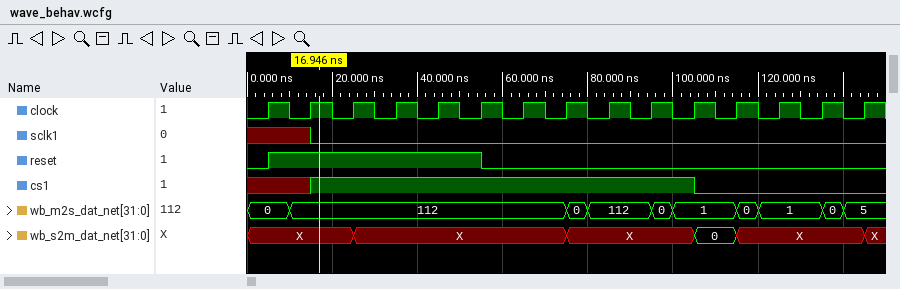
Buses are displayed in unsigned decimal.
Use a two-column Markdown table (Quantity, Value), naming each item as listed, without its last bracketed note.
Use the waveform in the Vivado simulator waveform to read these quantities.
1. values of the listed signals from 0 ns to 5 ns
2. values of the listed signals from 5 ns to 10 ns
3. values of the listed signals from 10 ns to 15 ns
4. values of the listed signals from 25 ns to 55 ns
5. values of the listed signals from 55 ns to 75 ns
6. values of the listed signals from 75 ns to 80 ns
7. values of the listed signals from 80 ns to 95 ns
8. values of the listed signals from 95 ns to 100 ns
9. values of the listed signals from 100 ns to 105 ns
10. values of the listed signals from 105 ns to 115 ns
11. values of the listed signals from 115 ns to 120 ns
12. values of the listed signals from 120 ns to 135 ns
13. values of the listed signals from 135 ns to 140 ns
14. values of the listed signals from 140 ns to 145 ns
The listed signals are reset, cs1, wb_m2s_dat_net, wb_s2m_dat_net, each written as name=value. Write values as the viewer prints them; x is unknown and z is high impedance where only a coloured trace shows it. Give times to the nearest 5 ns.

| Quantity | Value |
|---|---|
| values of the listed signals from 0 ns to 5 ns | reset=0, cs1=x, wb_m2s_dat_net=0, wb_s2m_dat_net=X |
| values of the listed signals from 5 ns to 10 ns | reset=1, cs1=x, wb_m2s_dat_net=0, wb_s2m_dat_net=X |
| values of the listed signals from 10 ns to 15 ns | reset=1, cs1=x, wb_m2s_dat_net=112, wb_s2m_dat_net=X |
| values of the listed signals from 25 ns to 55 ns | reset=1, cs1=1, wb_m2s_dat_net=112, wb_s2m_dat_net=X |
| values of the listed signals from 55 ns to 75 ns | reset=0, cs1=1, wb_m2s_dat_net=112, wb_s2m_dat_net=X |
| values of the listed signals from 75 ns to 80 ns | reset=0, cs1=1, wb_m2s_dat_net=0, wb_s2m_dat_net=X |
| values of the listed signals from 80 ns to 95 ns | reset=0, cs1=1, wb_m2s_dat_net=112, wb_s2m_dat_net=X |
| values of the listed signals from 95 ns to 100 ns | reset=0, cs1=1, wb_m2s_dat_net=0, wb_s2m_dat_net=X |
| values of the listed signals from 100 ns to 105 ns | reset=0, cs1=1, wb_m2s_dat_net=1, wb_s2m_dat_net=X |
| values of the listed signals from 105 ns to 115 ns | reset=0, cs1=0, wb_m2s_dat_net=1, wb_s2m_dat_net=0 |
| values of the listed signals from 115 ns to 120 ns | reset=0, cs1=0, wb_m2s_dat_net=0, wb_s2m_dat_net=X |
| values of the listed signals from 120 ns to 135 ns | reset=0, cs1=0, wb_m2s_dat_net=1, wb_s2m_dat_net=X |
| values of the listed signals from 135 ns to 140 ns | reset=0, cs1=0, wb_m2s_dat_net=0, wb_s2m_dat_net=X |
| values of the listed signals from 140 ns to 145 ns | reset=0, cs1=0, wb_m2s_dat_net=5, wb_s2m_dat_net=X |
